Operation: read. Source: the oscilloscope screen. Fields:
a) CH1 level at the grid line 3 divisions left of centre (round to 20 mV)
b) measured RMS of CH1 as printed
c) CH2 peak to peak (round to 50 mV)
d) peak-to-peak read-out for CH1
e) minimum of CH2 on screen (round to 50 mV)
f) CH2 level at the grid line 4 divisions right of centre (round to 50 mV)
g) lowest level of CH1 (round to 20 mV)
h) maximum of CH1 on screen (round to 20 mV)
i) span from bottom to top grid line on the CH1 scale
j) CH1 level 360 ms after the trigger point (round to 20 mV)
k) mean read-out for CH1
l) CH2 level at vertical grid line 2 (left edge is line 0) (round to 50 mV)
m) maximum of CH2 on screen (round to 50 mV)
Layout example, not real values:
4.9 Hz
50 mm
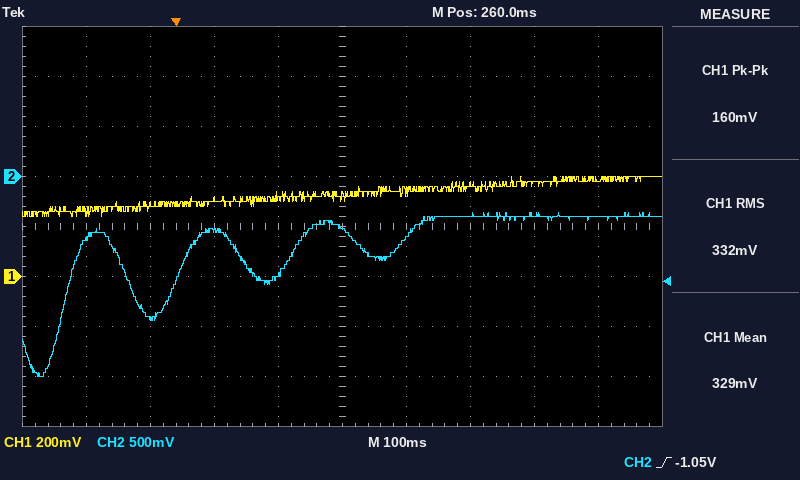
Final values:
280 mV
332 mV
1.65 V
160 mV
-2.00 V
-400 mV
240 mV
400 mV
1.6 V
340 mV
329 mV
-1.40 V
-350 mV
